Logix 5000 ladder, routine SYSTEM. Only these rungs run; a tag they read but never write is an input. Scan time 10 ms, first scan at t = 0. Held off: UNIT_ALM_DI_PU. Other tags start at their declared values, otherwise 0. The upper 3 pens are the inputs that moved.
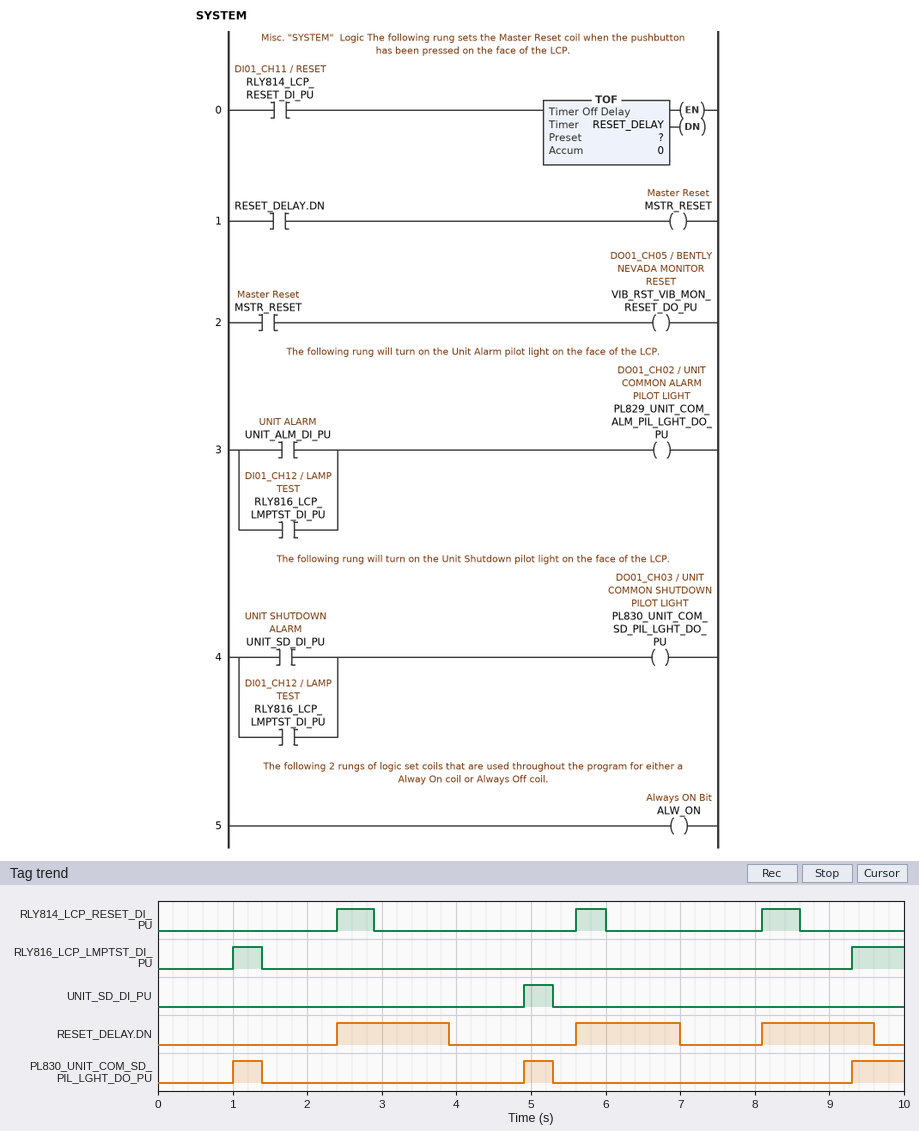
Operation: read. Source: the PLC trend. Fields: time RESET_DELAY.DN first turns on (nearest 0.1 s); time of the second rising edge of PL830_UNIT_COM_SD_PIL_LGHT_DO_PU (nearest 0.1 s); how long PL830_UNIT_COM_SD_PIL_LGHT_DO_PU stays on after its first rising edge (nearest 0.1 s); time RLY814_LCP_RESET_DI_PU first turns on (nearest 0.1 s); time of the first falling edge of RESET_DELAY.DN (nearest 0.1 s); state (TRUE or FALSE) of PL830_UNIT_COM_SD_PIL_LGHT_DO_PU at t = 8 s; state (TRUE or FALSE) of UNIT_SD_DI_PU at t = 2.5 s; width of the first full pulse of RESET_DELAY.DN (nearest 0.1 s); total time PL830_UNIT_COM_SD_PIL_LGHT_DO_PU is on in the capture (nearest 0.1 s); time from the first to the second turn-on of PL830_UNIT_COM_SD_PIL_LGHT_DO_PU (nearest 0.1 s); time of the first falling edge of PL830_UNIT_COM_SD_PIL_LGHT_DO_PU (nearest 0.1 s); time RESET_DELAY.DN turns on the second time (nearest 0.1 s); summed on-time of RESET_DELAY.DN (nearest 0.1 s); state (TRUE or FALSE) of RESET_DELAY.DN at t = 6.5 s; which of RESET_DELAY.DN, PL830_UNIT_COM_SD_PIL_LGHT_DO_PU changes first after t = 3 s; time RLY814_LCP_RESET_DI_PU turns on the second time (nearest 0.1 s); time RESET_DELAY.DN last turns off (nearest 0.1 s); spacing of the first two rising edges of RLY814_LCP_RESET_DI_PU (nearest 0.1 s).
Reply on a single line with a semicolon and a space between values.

2.4 s; 4.9 s; 0.4 s; 2.4 s; 3.9 s; FALSE; FALSE; 1.5 s; 1.5 s; 3.9 s; 1.4 s; 5.6 s; 4.4 s; TRUE; RESET_DELAY.DN; 5.6 s; 9.6 s; 3.2 s
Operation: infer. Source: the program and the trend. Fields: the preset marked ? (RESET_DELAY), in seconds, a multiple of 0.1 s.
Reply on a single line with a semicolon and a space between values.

1.0 s
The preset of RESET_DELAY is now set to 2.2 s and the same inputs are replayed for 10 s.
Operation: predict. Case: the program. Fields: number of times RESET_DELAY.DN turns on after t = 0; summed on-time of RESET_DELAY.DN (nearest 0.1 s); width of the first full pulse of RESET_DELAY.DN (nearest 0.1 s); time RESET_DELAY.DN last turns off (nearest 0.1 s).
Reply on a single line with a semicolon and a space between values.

2; 7.1 s; 2.7 s; 5.1 s
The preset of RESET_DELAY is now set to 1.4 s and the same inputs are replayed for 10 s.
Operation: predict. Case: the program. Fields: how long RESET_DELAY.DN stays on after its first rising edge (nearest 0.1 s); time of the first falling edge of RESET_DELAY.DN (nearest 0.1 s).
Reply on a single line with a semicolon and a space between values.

1.9 s; 4.3 s
